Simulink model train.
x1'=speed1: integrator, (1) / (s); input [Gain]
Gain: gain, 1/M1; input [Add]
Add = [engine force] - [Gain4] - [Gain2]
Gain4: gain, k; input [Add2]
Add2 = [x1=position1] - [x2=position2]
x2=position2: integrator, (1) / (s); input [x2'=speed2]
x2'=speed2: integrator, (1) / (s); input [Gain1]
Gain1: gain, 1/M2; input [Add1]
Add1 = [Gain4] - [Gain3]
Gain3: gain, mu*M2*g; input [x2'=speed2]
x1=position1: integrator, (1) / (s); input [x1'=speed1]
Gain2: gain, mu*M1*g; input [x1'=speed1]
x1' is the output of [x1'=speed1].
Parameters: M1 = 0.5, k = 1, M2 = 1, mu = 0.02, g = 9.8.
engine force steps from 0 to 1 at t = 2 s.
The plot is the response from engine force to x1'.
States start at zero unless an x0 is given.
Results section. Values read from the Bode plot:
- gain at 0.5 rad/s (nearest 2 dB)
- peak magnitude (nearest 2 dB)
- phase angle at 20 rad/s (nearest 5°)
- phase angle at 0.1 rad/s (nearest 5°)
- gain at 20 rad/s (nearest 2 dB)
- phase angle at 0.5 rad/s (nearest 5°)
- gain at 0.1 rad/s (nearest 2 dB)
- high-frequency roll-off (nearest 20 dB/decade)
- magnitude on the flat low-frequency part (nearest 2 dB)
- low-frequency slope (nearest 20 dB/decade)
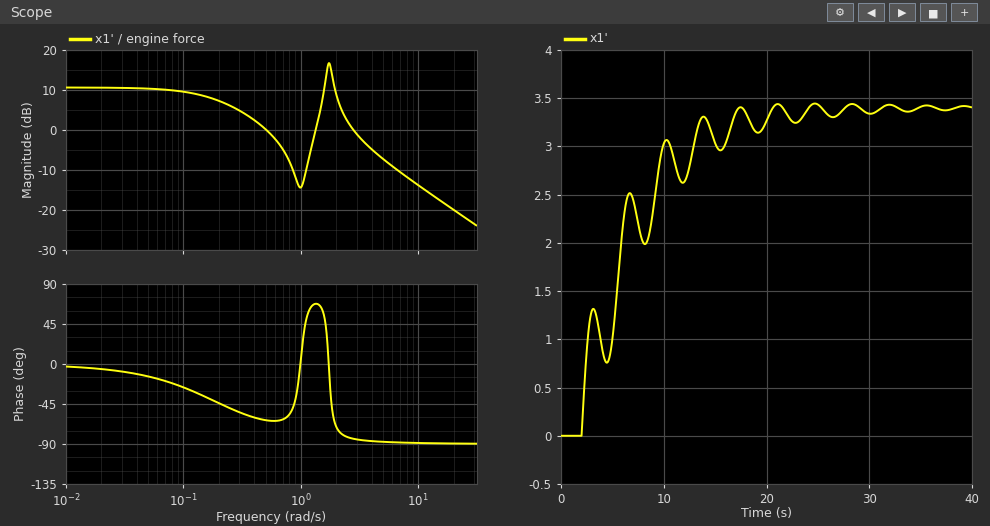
0 dB
16 dB
-90°
-25°
-20 dB
-65°
10 dB
-20 dB/decade
10 dB
0 dB/decade
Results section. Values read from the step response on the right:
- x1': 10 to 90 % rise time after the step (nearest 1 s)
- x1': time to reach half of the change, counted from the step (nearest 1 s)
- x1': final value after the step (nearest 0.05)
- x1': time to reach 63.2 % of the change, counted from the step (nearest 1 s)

8 s
4 s
3.40
4 s
